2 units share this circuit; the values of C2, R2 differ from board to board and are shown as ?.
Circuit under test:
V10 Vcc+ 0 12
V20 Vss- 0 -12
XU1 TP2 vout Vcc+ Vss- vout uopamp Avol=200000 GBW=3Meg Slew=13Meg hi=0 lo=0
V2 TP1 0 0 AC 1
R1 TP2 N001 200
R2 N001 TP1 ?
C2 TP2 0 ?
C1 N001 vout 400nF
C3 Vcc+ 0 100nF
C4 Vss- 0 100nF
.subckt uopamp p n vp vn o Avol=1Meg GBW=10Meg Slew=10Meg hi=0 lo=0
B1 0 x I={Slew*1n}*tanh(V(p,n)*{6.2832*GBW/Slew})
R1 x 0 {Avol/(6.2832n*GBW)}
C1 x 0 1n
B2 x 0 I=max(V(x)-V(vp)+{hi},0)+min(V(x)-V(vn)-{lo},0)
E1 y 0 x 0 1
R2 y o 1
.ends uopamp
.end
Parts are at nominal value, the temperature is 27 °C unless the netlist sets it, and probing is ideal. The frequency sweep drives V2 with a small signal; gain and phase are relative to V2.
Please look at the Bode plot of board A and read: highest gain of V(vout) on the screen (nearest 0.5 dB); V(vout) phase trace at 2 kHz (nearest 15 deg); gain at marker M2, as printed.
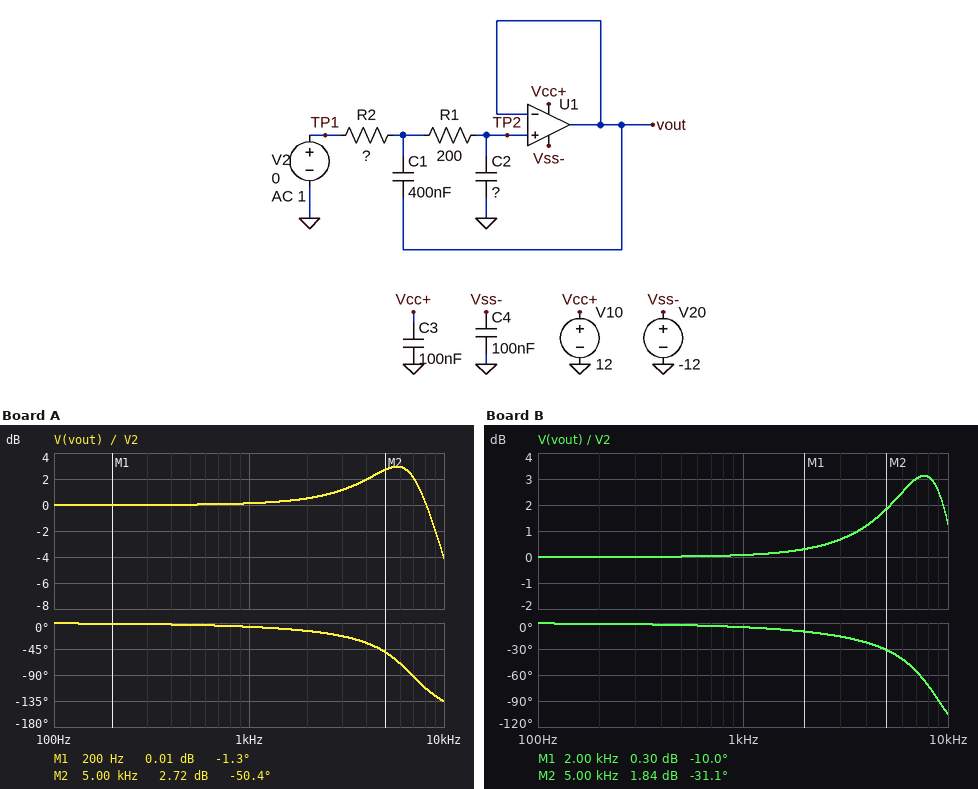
3.0 dB
-15 deg
2.72 dB
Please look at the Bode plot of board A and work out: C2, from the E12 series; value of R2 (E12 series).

56 nF
120 Ω
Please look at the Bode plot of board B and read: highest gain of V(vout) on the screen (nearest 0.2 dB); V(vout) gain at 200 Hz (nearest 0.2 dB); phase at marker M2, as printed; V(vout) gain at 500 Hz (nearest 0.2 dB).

3.2 dB
0 dB
-31.1 deg
0 dB
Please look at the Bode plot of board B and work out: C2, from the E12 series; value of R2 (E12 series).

47 nF
82 Ω
